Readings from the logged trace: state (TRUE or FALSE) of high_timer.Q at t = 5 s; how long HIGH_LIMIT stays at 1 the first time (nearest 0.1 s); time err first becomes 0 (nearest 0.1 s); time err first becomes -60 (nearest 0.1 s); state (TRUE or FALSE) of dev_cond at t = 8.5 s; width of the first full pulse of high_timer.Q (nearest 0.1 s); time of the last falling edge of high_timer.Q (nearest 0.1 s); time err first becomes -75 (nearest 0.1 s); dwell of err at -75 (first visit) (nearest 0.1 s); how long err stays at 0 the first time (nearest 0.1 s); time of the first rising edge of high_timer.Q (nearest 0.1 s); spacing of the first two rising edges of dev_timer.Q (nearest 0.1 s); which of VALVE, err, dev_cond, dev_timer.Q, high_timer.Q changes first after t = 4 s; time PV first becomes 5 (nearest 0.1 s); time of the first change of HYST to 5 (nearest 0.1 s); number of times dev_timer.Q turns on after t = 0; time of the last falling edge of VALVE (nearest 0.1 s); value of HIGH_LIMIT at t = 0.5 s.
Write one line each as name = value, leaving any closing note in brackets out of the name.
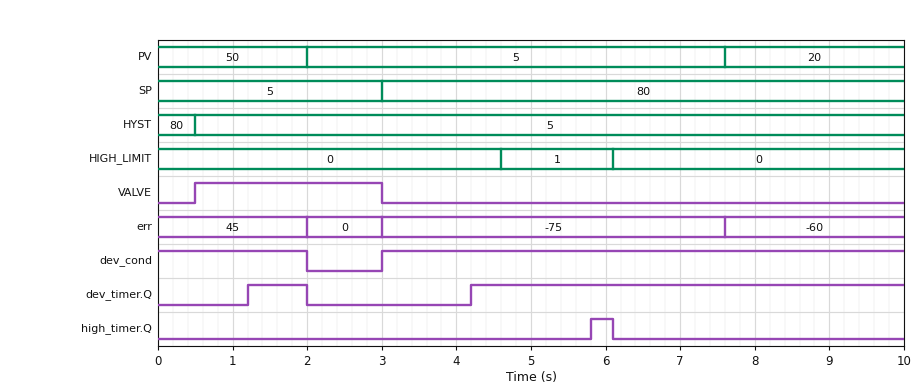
state (TRUE or FALSE) of high_timer.Q at t = 5 s = FALSE
how long HIGH_LIMIT stays at 1 the first time = 1.5 s
time err first becomes 0 = 2.0 s
time err first becomes -60 = 7.6 s
state (TRUE or FALSE) of dev_cond at t = 8.5 s = TRUE
width of the first full pulse of high_timer.Q = 0.3 s
time of the last falling edge of high_timer.Q = 6.1 s
time err first becomes -75 = 3.0 s
dwell of err at -75 (first visit) = 4.6 s
how long err stays at 0 the first time = 1.0 s
time of the first rising edge of high_timer.Q = 5.8 s
spacing of the first two rising edges of dev_timer.Q = 3.0 s
which of VALVE, err, dev_cond, dev_timer.Q, high_timer.Q changes first after t = 4 s = dev_timer.Q
time PV first becomes 5 = 2.0 s
time of the first change of HYST to 5 = 0.5 s
number of times dev_timer.Q turns on after t = 0 = 2
time of the last falling edge of VALVE = 3.0 s
value of HIGH_LIMIT at t = 0.5 s = 0
